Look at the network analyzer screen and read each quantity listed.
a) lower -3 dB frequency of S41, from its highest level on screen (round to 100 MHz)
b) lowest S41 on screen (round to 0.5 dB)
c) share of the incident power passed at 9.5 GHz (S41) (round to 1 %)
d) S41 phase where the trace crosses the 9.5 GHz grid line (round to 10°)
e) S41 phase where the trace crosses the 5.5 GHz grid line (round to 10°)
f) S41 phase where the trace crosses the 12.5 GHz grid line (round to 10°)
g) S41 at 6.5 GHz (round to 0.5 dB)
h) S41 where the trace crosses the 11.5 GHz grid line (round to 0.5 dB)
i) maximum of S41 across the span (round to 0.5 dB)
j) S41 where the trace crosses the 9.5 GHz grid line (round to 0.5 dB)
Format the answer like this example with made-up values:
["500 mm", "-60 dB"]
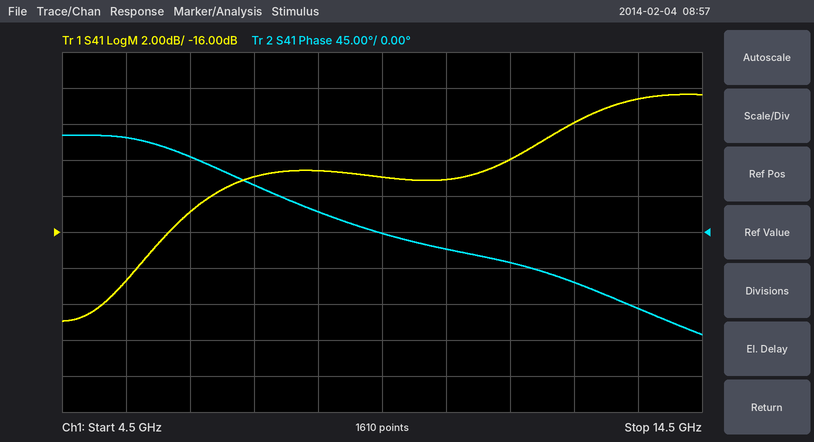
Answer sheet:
["11.8 GHz", "-21.0 dB", "5 %", "0°", "120°", "-60°", "-15.0 dB", "-12.0 dB", "-8.5 dB", "-13.0 dB"]
